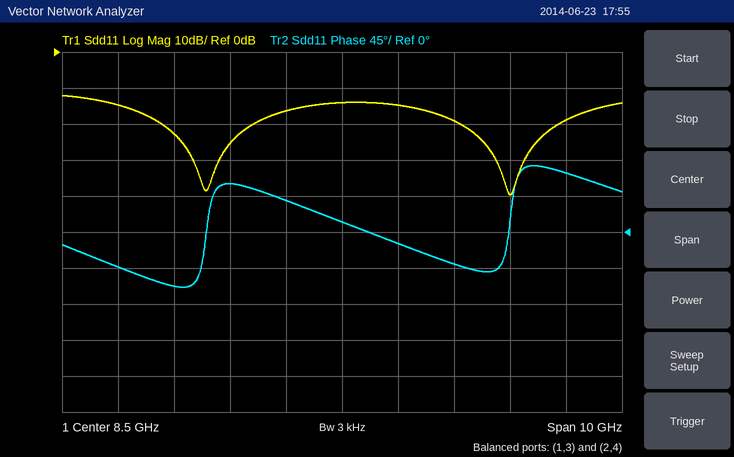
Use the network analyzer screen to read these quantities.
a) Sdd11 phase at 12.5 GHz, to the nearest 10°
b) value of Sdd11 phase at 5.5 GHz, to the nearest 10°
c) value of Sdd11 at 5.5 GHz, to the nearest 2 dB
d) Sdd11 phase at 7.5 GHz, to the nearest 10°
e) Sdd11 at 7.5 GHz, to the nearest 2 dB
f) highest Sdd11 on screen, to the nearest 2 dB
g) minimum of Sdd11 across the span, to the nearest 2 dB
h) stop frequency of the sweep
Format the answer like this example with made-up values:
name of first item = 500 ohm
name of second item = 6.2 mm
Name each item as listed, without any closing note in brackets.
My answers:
Sdd11 phase at 12.5 GHz, to the nearest 10° = 70°
value of Sdd11 phase at 5.5 GHz, to the nearest 10° = -70°
value of Sdd11 at 5.5 GHz, to the nearest 2 dB = -22 dB
Sdd11 phase at 7.5 GHz, to the nearest 10° = 40°
Sdd11 at 7.5 GHz, to the nearest 2 dB = -16 dB
highest Sdd11 on screen, to the nearest 2 dB = -12 dB
minimum of Sdd11 across the span, to the nearest 2 dB = -40 dB
stop frequency of the sweep = 13.5 GHz
